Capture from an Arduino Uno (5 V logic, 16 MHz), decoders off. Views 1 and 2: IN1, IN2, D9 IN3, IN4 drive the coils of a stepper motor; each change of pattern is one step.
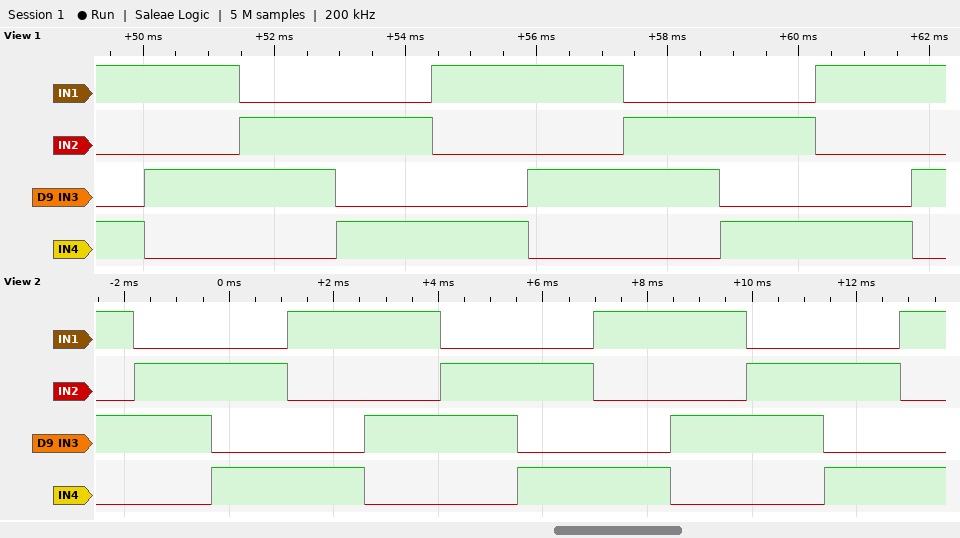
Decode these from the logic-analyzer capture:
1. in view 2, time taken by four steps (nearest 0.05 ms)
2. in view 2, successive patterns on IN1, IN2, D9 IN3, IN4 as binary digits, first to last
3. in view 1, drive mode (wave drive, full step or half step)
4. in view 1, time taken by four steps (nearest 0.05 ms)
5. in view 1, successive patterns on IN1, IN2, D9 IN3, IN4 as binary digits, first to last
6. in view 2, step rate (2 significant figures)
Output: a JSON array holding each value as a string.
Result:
["5.85 ms", "1010 0110 0101 1001 1010 0110 0101 1001 1010 0110 0101 1001", "full step", "5.85 ms", "1001 1010 0110 0101 1001 1010 0110 0101 1001 1010", "680 steps/s"]
